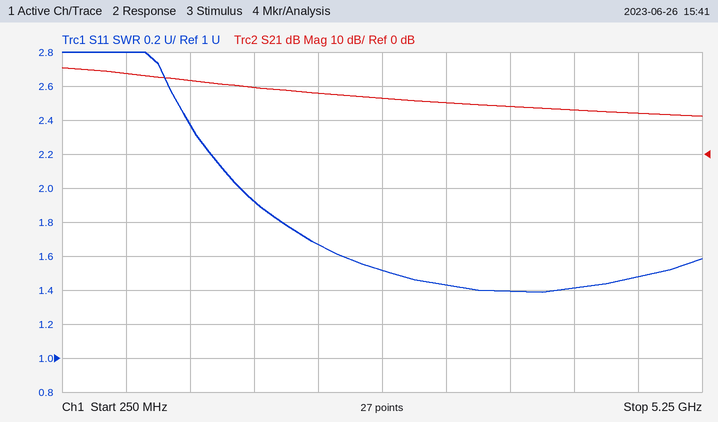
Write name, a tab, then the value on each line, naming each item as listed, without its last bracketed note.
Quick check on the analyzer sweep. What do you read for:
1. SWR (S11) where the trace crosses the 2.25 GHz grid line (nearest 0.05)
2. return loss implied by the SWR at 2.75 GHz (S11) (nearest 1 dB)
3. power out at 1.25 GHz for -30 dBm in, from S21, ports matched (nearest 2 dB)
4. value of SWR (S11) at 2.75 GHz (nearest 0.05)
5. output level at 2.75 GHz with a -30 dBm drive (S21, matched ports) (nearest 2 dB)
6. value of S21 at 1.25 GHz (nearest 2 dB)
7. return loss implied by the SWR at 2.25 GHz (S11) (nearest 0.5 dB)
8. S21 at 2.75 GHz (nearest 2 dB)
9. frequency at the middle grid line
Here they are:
SWR (S11) where the trace crosses the 2.25 GHz grid line	1.65
return loss implied by the SWR at 2.75 GHz (S11)	14 dB
power out at 1.25 GHz for -30 dBm in, from S21, ports matched	-8 dBm
value of SWR (S11) at 2.75 GHz	1.50
output level at 2.75 GHz with a -30 dBm drive (S21, matched ports)	-14 dBm
value of S21 at 1.25 GHz	22 dB
return loss implied by the SWR at 2.25 GHz (S11)	12.0 dB
S21 at 2.75 GHz	16 dB
frequency at the middle grid line	2.75 GHz
